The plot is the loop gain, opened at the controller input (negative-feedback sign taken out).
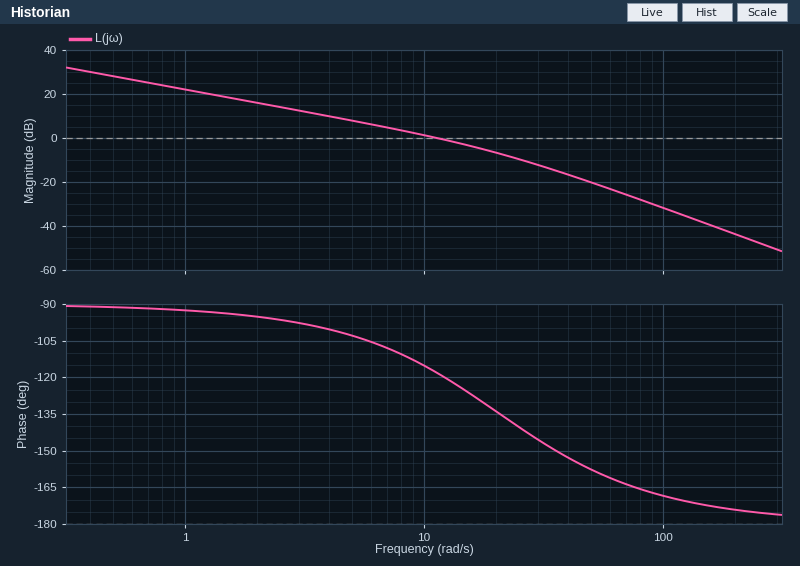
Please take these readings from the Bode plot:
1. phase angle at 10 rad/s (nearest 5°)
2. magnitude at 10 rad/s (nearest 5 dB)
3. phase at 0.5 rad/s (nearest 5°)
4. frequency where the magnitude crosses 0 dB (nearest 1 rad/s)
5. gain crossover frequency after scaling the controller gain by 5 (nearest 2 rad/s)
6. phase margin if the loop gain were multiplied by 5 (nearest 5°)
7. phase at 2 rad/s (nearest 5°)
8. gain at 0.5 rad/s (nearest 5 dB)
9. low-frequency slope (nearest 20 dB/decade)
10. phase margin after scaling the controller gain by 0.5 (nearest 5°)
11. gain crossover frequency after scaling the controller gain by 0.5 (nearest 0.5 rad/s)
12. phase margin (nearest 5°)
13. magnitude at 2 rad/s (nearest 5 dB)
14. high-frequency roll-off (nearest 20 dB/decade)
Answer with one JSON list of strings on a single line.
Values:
["-115°", "0 dB", "-90°", "11 rad/s", "34 rad/s", "30°", "-95°", "30 dB", "-20 dB/decade", "75°", "6.0 rad/s", "60°", "15 dB", "-40 dB/decade"]
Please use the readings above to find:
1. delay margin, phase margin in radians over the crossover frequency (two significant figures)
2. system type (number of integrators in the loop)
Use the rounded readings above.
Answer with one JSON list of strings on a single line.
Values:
["0.095 s", "1"]
